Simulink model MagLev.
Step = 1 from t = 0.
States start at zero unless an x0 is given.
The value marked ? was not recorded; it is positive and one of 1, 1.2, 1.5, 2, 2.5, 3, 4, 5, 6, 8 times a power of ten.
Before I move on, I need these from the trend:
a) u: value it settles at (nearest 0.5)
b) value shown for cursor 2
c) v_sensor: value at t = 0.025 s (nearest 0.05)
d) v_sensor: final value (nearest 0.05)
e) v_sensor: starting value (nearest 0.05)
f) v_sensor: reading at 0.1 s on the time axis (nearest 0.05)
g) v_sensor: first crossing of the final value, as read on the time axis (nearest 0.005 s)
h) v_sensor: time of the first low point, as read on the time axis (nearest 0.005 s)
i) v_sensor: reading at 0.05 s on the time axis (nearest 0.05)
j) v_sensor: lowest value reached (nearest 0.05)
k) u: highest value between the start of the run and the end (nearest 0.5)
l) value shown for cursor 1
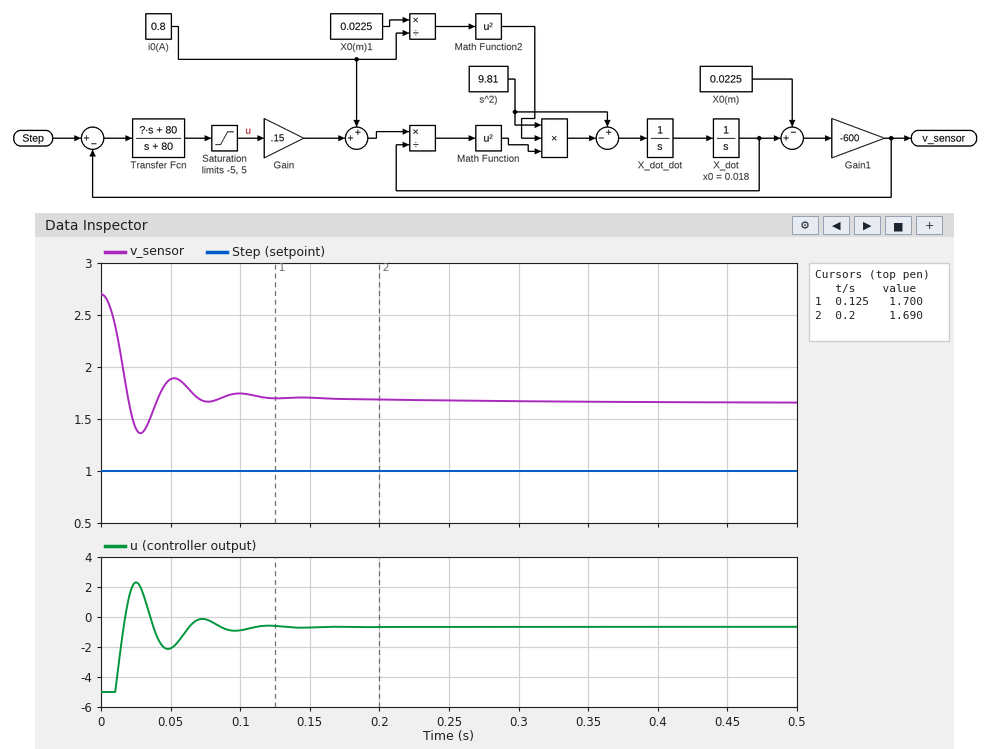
-0.5
1.690
1.40
1.65
2.70
1.75
0.020 s
0.030 s
1.90
1.35
2.5
1.700
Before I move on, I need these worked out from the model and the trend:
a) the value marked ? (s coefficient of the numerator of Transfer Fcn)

8
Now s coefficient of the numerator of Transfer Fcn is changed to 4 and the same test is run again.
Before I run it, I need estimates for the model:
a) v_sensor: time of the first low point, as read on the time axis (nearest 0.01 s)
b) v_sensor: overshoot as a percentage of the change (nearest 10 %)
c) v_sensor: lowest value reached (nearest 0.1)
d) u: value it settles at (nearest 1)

0.04 s
50 %
1.1
-1
